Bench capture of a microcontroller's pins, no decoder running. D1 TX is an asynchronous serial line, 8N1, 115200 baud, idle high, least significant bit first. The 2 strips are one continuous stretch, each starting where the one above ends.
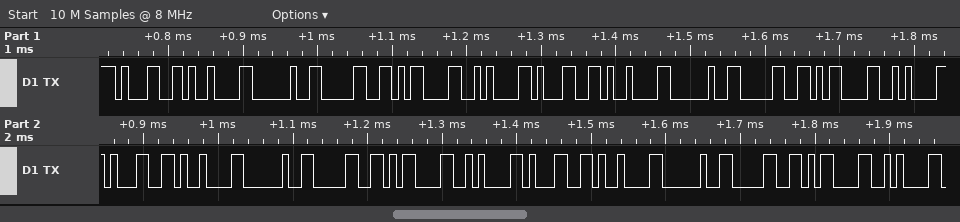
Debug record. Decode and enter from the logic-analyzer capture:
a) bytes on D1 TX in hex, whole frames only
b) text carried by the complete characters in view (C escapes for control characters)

31 09 20 30 0D 0A 31 09 20 30 0D 0A 31 09 20 30 0D 0A 31 09 20 30 0D 0A
"1\t 0\r\n1\t 0\r\n1\t 0\r\n1\t 0\r\n"
